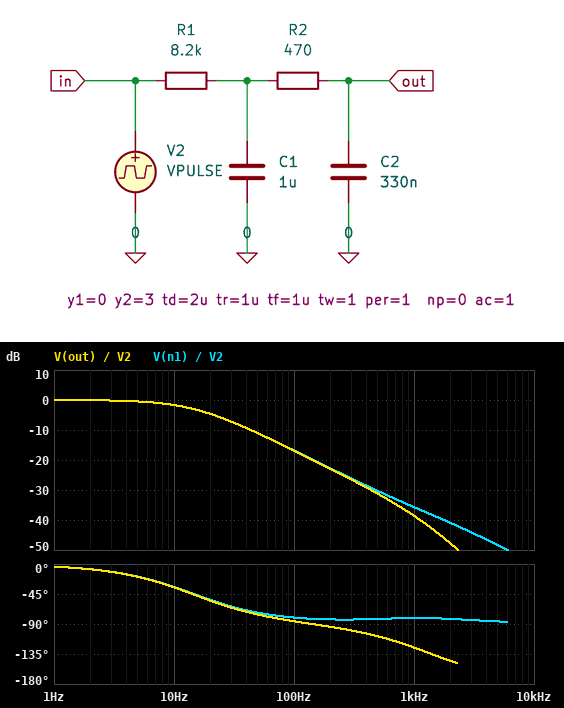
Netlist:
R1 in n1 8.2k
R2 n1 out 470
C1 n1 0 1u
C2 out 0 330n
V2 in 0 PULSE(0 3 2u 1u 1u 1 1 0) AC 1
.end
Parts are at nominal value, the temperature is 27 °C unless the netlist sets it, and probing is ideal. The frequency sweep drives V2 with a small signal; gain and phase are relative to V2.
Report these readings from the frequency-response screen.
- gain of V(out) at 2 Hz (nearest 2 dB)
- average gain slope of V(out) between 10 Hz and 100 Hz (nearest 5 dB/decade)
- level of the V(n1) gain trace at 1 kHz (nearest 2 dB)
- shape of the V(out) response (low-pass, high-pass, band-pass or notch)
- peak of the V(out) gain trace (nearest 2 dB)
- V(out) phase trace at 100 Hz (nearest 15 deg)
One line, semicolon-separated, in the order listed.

0 dB; -15 dB/decade; -36 dB; low-pass; 0 dB; -90 deg
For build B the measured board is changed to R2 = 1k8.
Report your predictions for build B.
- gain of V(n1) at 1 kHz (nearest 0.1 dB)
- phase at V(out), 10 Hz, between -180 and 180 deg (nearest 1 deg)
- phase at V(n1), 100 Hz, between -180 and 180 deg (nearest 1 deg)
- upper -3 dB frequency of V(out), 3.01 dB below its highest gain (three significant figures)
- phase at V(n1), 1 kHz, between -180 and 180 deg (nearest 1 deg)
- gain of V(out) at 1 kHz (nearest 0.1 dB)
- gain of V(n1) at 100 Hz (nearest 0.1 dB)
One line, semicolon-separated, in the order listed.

-34.5 dB; -36 deg; -77 deg; 14.4 Hz; -84 deg; -46.2 dB; -16.7 dB
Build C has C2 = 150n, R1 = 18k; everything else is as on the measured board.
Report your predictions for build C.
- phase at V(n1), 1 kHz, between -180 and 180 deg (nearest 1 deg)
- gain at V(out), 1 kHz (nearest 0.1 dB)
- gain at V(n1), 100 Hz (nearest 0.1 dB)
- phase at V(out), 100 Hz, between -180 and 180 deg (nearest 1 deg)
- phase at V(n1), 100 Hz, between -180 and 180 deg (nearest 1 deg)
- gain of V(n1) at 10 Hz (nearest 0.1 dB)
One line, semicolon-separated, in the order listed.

-87 deg; -42.9 dB; -22.3 dB; -88 deg; -85 deg; -4.3 dB
